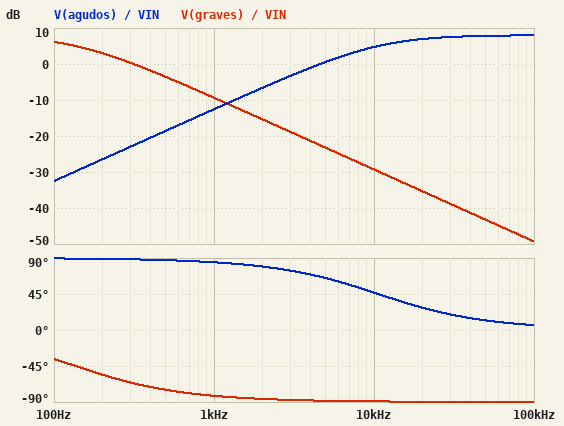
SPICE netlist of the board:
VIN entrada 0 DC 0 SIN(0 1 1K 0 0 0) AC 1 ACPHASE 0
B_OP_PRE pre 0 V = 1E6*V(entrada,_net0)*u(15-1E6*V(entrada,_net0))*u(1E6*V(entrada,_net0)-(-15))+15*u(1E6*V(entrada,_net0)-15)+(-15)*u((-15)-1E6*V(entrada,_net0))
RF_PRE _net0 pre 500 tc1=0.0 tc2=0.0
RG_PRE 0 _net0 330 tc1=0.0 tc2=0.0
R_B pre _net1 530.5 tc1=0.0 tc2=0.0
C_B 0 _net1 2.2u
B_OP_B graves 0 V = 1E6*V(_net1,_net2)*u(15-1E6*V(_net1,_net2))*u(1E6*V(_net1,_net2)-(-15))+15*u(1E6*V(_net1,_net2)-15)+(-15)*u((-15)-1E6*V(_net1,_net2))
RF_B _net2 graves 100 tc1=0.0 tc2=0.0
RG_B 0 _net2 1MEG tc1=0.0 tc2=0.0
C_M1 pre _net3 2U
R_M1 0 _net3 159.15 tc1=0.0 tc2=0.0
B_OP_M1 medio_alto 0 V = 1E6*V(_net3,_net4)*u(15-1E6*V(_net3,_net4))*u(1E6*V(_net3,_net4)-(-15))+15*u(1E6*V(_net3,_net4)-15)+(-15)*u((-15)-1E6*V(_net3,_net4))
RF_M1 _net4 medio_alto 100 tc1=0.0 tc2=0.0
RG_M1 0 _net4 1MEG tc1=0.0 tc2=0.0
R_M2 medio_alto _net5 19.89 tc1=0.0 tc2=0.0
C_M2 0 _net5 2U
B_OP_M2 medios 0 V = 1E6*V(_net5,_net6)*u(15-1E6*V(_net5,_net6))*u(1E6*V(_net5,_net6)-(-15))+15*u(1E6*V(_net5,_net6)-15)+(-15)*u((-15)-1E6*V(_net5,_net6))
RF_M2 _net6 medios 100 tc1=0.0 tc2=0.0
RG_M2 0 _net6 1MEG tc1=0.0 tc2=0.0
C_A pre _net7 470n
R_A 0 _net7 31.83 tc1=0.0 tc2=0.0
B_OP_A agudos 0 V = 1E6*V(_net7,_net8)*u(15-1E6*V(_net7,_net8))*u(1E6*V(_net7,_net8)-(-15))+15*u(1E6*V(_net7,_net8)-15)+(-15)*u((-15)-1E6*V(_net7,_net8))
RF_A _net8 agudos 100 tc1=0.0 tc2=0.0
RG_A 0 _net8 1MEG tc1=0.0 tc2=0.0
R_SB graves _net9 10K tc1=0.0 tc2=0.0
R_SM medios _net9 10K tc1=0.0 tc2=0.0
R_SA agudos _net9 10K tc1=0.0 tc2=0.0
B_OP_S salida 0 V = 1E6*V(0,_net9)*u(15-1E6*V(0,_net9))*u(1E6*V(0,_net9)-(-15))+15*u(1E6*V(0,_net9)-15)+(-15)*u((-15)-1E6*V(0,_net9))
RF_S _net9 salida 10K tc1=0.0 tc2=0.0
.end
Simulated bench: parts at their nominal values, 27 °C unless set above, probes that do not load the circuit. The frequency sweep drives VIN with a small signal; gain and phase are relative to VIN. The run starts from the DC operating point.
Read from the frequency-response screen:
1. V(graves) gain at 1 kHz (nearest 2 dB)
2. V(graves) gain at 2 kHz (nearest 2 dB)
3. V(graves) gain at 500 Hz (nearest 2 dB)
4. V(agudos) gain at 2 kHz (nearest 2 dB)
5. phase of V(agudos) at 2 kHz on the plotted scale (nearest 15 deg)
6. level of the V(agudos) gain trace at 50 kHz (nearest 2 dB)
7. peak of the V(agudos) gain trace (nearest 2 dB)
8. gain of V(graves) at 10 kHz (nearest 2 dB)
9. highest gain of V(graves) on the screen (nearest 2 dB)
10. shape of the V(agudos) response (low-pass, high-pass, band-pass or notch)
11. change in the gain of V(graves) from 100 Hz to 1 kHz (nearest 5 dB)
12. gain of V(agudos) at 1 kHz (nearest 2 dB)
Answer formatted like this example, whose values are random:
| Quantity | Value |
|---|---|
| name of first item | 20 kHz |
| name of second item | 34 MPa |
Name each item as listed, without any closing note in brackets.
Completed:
| Quantity | Value |
|---|---|
| V(graves) gain at 1 kHz | -10 dB |
| V(graves) gain at 2 kHz | -16 dB |
| V(graves) gain at 500 Hz | -4 dB |
| V(agudos) gain at 2 kHz | -6 dB |
| phase of V(agudos) at 2 kHz on the plotted scale | 75 deg |
| level of the V(agudos) gain trace at 50 kHz | 8 dB |
| peak of the V(agudos) gain trace | 8 dB |
| gain of V(graves) at 10 kHz | -30 dB |
| highest gain of V(graves) on the screen | 6 dB |
| shape of the V(agudos) response | high-pass |
| change in the gain of V(graves) from 100 Hz to 1 kHz | -15 dB |
| gain of V(agudos) at 1 kHz | -12 dB |
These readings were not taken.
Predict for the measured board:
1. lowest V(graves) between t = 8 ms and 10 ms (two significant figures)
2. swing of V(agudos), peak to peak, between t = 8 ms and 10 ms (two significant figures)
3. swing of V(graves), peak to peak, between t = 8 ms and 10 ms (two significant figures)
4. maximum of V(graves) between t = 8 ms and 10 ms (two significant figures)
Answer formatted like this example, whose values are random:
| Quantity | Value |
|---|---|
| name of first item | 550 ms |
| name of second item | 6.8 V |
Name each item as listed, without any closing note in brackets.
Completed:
| Quantity | Value |
|---|---|
| lowest V(graves) between t = 8 ms and 10 ms | -340 mV |
| swing of V(agudos), peak to peak, between t = 8 ms and 10 ms | 470 mV |
| swing of V(graves), peak to peak, between t = 8 ms and 10 ms | 680 mV |
| maximum of V(graves) between t = 8 ms and 10 ms | 340 mV |
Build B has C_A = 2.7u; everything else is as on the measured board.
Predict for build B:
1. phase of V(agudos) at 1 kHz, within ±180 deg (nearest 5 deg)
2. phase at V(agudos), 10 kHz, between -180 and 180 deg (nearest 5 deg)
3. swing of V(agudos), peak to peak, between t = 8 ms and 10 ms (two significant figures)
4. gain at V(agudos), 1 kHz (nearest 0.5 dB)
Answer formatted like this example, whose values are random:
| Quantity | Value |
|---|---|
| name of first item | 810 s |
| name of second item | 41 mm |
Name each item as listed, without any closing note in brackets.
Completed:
| Quantity | Value |
|---|---|
| phase of V(agudos) at 1 kHz, within ±180 deg | 60 deg |
| phase at V(agudos), 10 kHz, between -180 and 180 deg | 10 deg |
| swing of V(agudos), peak to peak, between t = 8 ms and 10 ms | 2.4 V |
| gain at V(agudos), 1 kHz | 1.5 dB |
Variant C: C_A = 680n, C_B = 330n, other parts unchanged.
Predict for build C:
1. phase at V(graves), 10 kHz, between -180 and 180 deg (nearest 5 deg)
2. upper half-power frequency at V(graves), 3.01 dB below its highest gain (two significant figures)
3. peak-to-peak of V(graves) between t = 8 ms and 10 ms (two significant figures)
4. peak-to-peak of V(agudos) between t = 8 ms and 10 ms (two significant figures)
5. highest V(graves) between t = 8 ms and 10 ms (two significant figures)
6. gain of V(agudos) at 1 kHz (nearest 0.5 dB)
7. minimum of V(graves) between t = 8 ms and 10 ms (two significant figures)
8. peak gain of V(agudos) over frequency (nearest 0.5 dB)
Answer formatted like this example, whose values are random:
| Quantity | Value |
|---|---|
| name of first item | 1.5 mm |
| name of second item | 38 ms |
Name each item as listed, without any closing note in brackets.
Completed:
| Quantity | Value |
|---|---|
| phase at V(graves), 10 kHz, between -180 and 180 deg | -85 deg |
| upper half-power frequency at V(graves), 3.01 dB below its highest gain | 910 Hz |
| peak-to-peak of V(graves) between t = 8 ms and 10 ms | 3.4 V |
| peak-to-peak of V(agudos) between t = 8 ms and 10 ms | 680 mV |
| highest V(graves) between t = 8 ms and 10 ms | 1.7 V |
| gain of V(agudos) at 1 kHz | -9.5 dB |
| minimum of V(graves) between t = 8 ms and 10 ms | -1.7 V |
| peak gain of V(agudos) over frequency | 8.0 dB |
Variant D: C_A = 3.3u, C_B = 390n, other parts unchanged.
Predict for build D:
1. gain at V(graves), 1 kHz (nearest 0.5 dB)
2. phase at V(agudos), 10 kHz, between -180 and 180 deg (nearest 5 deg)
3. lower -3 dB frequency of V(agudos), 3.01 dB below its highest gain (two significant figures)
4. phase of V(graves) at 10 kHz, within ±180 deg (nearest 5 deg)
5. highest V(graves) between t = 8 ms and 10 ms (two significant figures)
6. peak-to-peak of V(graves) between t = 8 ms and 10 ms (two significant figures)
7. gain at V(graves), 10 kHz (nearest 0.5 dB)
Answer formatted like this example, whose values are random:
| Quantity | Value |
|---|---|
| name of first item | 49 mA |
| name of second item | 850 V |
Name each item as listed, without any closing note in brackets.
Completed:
| Quantity | Value |
|---|---|
| gain at V(graves), 1 kHz | 3.5 dB |
| phase at V(agudos), 10 kHz, between -180 and 180 deg | 10 deg |
| lower -3 dB frequency of V(agudos), 3.01 dB below its highest gain | 1.5 kHz |
| phase of V(graves) at 10 kHz, within ±180 deg | -85 deg |
| highest V(graves) between t = 8 ms and 10 ms | 1.5 V |
| peak-to-peak of V(graves) between t = 8 ms and 10 ms | 3.1 V |
| gain at V(graves), 10 kHz | -14.5 dB |
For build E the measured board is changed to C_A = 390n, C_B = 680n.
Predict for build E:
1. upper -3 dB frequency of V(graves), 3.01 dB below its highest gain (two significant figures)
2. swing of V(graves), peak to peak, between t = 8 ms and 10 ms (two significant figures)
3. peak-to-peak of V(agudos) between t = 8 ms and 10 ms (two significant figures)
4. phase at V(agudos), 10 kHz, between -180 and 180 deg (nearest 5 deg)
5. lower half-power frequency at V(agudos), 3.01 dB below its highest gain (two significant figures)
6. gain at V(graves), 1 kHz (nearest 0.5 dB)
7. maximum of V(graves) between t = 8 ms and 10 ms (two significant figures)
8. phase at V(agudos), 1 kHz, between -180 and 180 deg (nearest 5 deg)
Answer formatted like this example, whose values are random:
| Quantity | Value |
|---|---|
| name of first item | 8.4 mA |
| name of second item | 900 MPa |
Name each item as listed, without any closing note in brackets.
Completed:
| Quantity | Value |
|---|---|
| upper -3 dB frequency of V(graves), 3.01 dB below its highest gain | 440 Hz |
| swing of V(graves), peak to peak, between t = 8 ms and 10 ms | 2.0 V |
| peak-to-peak of V(agudos) between t = 8 ms and 10 ms | 390 mV |
| phase at V(agudos), 10 kHz, between -180 and 180 deg | 50 deg |
| lower half-power frequency at V(agudos), 3.01 dB below its highest gain | 13 kHz |
| gain at V(graves), 1 kHz | 0 dB |
| maximum of V(graves) between t = 8 ms and 10 ms | 1.0 V |
| phase at V(agudos), 1 kHz, between -180 and 180 deg | 85 deg |
